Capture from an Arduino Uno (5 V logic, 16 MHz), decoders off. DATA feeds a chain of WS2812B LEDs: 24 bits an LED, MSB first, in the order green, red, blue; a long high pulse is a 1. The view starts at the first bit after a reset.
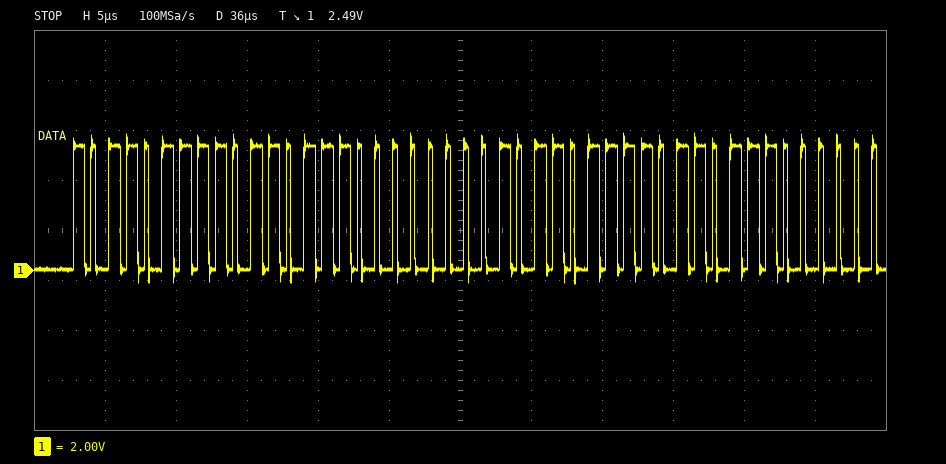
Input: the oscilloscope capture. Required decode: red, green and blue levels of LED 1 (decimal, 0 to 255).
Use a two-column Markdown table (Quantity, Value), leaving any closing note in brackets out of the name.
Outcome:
| Quantity | Value |
|---|---|
| red, green and blue levels of LED 1 | 183, 183, 0 |
